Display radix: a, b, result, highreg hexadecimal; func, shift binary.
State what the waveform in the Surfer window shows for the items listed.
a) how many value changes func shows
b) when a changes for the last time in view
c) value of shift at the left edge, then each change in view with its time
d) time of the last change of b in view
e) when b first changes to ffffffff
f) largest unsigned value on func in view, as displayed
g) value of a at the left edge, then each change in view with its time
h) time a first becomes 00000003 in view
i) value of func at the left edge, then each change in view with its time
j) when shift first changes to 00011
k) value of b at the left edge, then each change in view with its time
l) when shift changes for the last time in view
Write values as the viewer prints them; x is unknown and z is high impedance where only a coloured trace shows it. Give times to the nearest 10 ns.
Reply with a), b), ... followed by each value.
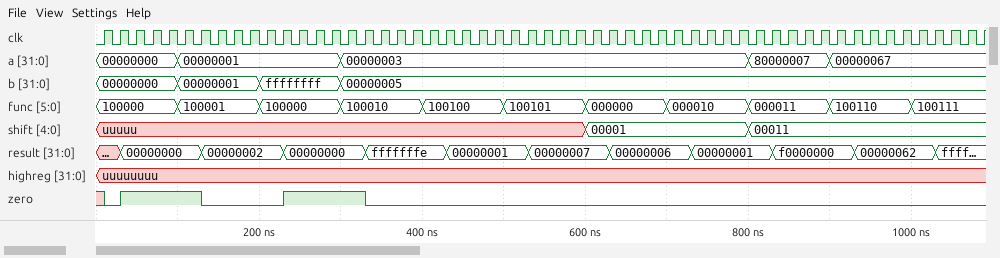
a) 10
b) 900 ns
c) uuuuu, 00001 at 600 ns, 00011 at 800 ns
d) 300 ns
e) 200 ns
f) 100111
g) 00000000, 00000001 at 100 ns, 00000003 at 300 ns, 80000007 at 800 ns, 00000067 at 900 ns
h) 300 ns
i) 100000, 100001 at 100 ns, 100000 at 200 ns, 100010 at 300 ns, 100100 at 400 ns, 100101 at 500 ns, 000000 at 600 ns, 000010 at 700 ns, 000011 at 800 ns, 100110 at 900 ns, 100111 at 1000 ns
j) 800 ns
k) 00000000, 00000001 at 100 ns, ffffffff at 200 ns, 00000005 at 300 ns
l) 800 ns
